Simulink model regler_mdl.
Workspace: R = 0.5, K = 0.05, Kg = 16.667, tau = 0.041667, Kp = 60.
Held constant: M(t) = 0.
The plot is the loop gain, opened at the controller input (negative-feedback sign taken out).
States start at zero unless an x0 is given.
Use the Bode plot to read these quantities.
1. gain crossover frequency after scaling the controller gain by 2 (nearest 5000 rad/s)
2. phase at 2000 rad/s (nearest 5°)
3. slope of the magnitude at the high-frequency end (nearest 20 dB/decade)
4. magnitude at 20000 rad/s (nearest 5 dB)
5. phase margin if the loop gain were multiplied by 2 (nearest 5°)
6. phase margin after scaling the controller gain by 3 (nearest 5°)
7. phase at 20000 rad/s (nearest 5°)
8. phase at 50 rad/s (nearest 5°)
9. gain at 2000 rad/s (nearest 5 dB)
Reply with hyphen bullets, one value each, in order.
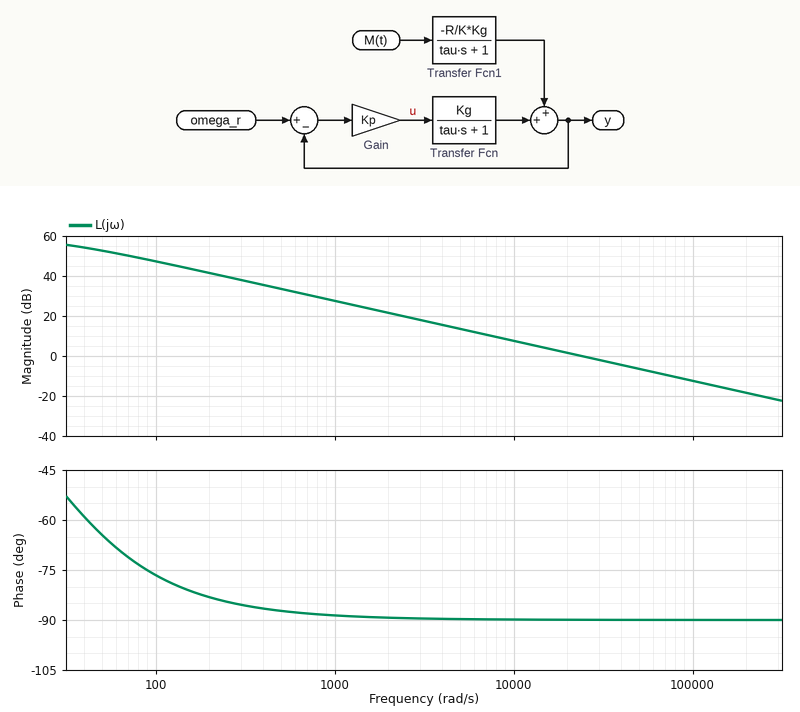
- 50000 rad/s
- -90°
- -20 dB/decade
- 0 dB
- 90°
- 90°
- -90°
- -65°
- 20 dB
